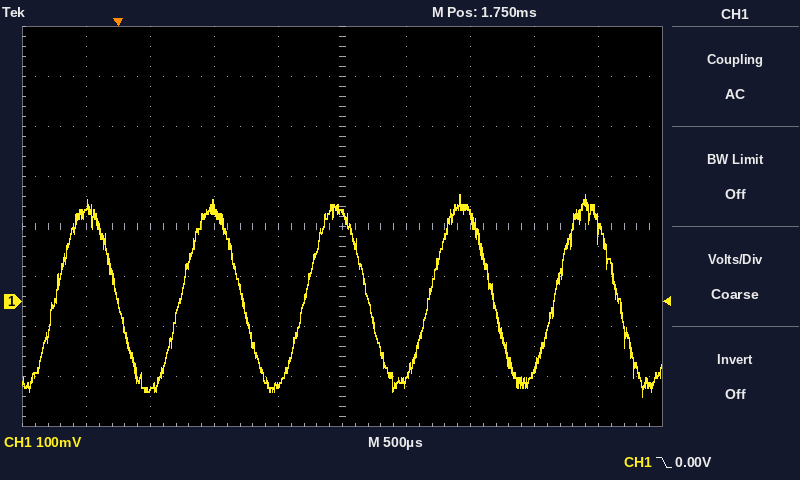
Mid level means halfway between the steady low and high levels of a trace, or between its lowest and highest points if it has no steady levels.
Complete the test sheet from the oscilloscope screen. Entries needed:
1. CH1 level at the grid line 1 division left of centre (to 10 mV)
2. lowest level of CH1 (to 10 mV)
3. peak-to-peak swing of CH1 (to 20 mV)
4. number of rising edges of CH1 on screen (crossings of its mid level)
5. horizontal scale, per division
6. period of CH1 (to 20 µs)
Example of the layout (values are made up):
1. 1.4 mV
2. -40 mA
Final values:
1. -170 mV
2. -190 mV
3. 400 mV
4. 5
5. 500 µs
6. 980 µs
